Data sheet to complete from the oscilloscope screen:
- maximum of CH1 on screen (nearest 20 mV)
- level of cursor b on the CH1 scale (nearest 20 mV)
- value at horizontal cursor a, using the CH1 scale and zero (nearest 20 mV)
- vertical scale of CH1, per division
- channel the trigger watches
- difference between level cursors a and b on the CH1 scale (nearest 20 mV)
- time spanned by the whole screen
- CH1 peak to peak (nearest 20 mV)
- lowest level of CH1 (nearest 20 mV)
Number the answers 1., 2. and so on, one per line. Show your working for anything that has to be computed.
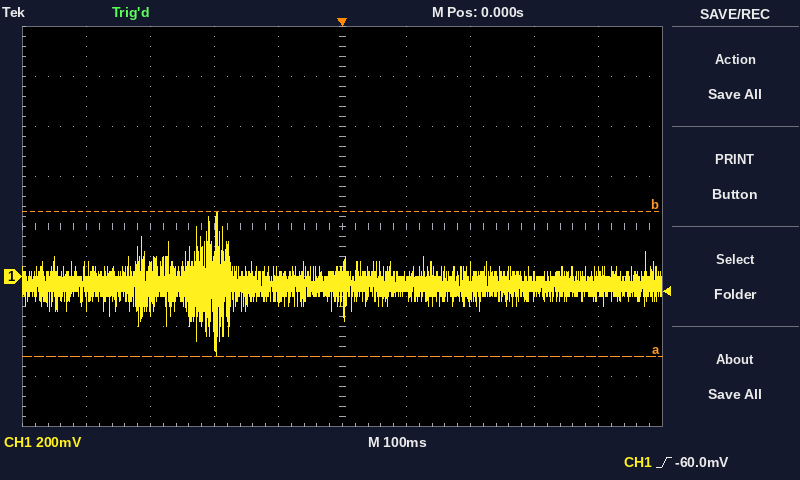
1. 260 mV
2. 260 mV
3. -320 mV
4. 200 mV
5. CH1
6. 580 mV
7. 1 s
8. 260 mV − (-320 mV) = 580 mV
9. -320 mV
